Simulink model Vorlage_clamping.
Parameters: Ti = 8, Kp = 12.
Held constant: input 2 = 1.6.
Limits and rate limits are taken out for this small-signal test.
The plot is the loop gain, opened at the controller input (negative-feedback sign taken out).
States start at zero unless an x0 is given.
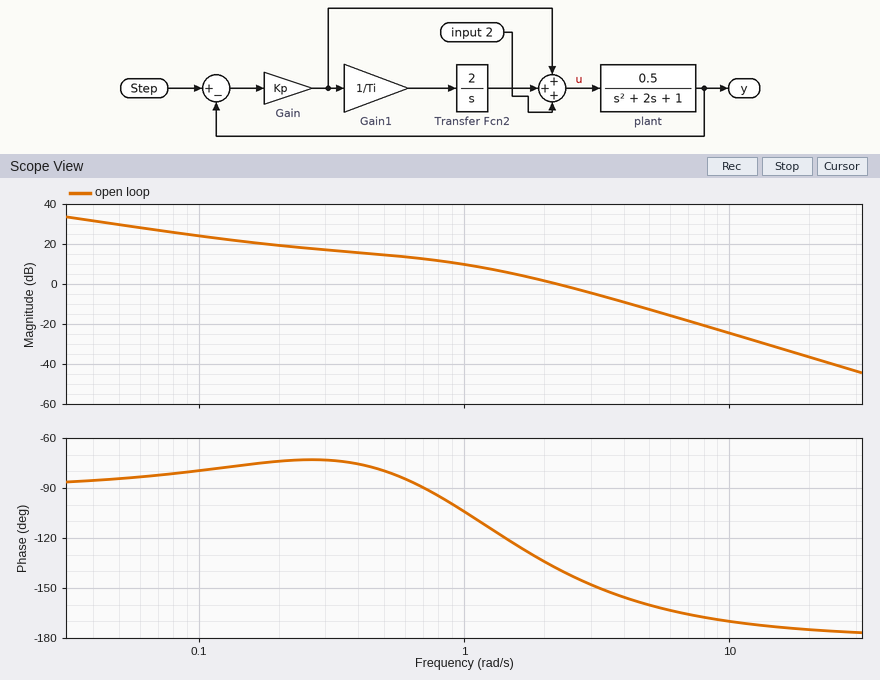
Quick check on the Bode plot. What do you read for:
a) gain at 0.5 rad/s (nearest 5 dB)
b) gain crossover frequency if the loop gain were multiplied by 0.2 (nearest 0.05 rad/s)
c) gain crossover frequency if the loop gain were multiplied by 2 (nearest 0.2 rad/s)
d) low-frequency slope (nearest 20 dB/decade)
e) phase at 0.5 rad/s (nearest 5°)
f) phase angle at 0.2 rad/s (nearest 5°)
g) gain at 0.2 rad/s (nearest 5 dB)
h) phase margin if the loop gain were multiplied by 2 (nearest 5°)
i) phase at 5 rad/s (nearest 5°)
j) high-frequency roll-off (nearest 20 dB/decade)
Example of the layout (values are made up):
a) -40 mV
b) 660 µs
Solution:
a) 15 dB
b) 0.55 rad/s
c) 3.4 rad/s
d) -20 dB/decade
e) -80°
f) -75°
g) 20 dB
h) 30°
i) -160°
j) -40 dB/decade
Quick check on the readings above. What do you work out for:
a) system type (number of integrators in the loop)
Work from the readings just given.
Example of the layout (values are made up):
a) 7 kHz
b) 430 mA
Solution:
a) 1
